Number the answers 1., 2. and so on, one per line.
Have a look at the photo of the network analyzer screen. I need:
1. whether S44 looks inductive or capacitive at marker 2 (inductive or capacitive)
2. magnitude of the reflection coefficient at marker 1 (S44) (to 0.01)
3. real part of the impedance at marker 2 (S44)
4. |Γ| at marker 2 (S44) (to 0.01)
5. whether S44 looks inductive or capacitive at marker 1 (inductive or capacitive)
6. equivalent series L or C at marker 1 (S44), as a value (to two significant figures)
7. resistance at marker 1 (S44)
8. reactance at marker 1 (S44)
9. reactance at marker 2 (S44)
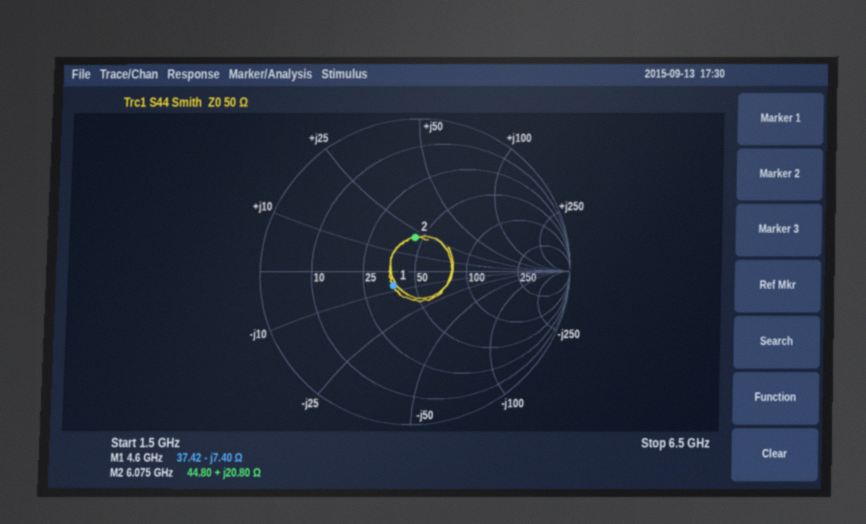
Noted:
1. inductive
2. 0.17
3. 44.80 Ω
4. 0.22
5. capacitive
6. 4.7 pF
7. 37.42 Ω
8. -7.40 Ω
9. +20.80 Ω
